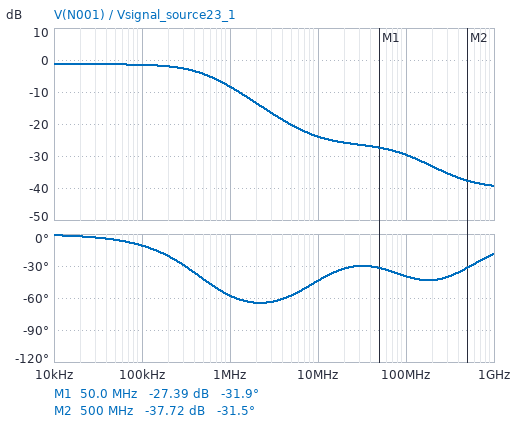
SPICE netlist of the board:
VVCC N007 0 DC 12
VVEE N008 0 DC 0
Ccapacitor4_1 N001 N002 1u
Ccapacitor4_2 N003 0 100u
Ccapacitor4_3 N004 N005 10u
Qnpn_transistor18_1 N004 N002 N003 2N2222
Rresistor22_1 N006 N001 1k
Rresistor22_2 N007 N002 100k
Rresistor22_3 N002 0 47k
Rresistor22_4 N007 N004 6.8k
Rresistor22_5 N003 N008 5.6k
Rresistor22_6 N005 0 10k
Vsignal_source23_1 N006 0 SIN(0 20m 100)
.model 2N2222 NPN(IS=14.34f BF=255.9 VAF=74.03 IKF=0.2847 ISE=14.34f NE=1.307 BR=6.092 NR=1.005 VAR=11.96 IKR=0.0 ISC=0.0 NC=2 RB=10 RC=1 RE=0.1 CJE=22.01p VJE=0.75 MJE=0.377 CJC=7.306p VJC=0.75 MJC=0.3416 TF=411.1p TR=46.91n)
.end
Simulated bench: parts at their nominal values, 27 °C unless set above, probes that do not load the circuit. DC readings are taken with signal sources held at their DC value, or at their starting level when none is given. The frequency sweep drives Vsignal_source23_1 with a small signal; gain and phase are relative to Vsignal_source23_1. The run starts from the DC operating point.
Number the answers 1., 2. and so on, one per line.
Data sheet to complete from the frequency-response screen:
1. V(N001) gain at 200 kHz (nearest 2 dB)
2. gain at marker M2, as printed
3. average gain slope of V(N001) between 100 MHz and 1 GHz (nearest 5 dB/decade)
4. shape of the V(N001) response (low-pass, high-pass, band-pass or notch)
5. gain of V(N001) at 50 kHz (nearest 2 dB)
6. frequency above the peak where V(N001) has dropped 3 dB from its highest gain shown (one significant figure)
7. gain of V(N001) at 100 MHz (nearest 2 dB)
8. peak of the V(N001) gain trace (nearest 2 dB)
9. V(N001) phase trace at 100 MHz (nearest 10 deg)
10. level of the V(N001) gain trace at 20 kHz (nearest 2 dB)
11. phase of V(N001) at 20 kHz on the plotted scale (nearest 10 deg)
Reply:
1. -2 dB
2. -37.72 dB
3. -10 dB/decade
4. low-pass
5. -2 dB
6. 500 kHz
7. -30 dB
8. -2 dB
9. -40 deg
10. -2 dB
11. 0 deg
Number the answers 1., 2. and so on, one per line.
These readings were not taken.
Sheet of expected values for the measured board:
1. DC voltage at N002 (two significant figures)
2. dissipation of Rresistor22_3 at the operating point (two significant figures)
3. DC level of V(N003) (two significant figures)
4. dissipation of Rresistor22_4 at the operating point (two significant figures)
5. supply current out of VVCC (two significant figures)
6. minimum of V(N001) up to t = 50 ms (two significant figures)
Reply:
1. 3.7 V
2. 290 µW
3. 3.1 V
4. 2.0 mW
5. 630 µA
6. -18 mV
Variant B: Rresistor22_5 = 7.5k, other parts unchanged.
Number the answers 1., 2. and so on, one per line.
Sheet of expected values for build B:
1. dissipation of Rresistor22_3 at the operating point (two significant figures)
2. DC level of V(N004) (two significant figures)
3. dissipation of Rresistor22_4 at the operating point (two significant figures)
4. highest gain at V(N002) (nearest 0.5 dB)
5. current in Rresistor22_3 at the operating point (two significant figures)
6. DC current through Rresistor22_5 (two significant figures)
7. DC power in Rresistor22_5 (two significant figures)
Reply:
1. 300 µW
2. 9.2 V
3. 1.2 mW
4. -1.0 dB
5. 80 µA
6. 420 µA
7. 1.3 mW
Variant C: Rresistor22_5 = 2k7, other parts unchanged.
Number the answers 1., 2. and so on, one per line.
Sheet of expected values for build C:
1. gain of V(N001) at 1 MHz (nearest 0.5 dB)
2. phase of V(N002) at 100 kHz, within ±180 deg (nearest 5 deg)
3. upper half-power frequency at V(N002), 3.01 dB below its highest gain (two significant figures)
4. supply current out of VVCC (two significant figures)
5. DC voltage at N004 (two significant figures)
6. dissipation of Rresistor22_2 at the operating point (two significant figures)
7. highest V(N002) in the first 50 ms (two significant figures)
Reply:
1. -15.5 dB
2. -25 deg
3. 220 kHz
4. 1.2 mA
5. 4.6 V
6. 710 µW
7. 3.6 V
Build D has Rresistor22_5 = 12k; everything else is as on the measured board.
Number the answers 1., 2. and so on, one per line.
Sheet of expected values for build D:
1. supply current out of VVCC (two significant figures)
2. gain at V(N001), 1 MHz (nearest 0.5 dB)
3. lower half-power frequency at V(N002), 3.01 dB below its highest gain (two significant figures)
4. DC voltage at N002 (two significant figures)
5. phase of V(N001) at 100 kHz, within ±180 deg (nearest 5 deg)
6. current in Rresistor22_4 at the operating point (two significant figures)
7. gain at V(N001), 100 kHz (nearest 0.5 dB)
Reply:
1. 340 µA
2. -4.0 dB
3. 15 Hz
4. 3.8 V
5. -5 deg
6. 260 µA
7. -1.0 dB
